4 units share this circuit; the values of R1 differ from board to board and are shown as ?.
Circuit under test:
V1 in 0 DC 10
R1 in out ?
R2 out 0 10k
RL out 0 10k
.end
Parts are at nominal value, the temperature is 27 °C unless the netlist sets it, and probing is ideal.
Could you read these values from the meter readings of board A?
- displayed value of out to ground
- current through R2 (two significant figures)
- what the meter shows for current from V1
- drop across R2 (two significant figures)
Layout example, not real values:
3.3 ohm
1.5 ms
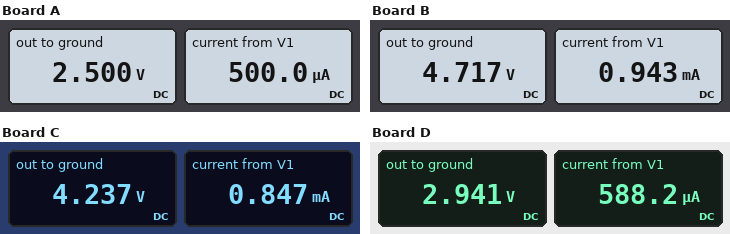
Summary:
2.500 V
250 µA
500.0 µA
2.5 V
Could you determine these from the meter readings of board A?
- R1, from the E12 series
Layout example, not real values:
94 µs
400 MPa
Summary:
15 kΩ
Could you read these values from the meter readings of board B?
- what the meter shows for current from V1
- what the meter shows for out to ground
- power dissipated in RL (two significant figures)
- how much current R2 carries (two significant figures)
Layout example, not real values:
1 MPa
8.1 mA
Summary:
0.943 mA
4.717 V
2.2 mW
470 µA
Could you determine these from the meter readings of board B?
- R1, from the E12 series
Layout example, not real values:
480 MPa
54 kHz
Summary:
5.6 kΩ
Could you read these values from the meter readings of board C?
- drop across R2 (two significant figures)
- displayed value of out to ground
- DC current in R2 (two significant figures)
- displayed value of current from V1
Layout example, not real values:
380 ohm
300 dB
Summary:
4.2 V
4.237 V
420 µA
0.847 mA
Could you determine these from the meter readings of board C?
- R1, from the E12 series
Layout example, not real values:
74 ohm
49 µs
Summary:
6.8 kΩ
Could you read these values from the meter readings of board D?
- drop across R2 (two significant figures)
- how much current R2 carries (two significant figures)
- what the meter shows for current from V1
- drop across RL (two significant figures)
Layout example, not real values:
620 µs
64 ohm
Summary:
2.9 V
290 µA
588.2 µA
2.9 V
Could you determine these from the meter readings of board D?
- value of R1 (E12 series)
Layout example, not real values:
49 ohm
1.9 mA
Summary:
12 kΩ
